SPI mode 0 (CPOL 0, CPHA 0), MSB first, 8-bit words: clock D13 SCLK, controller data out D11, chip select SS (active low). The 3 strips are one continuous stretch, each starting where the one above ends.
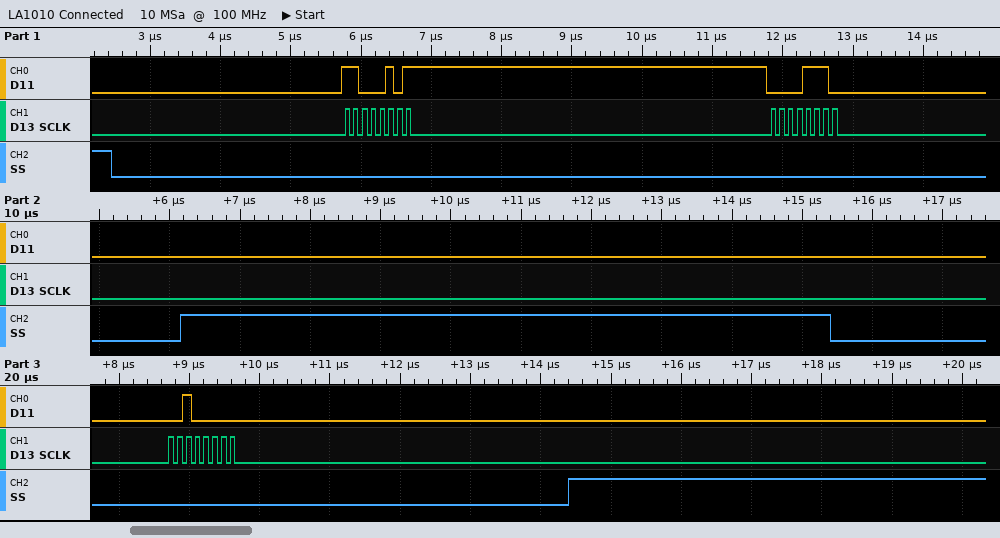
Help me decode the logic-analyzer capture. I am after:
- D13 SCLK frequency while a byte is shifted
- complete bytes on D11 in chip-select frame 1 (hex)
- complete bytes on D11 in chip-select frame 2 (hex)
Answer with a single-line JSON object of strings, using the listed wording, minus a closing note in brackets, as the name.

{"D13 SCLK frequency while a byte is shifted": "8 MHz", "complete bytes on D11 in chip-select frame 1": "C5 0E", "complete bytes on D11 in chip-select frame 2": "20"}
